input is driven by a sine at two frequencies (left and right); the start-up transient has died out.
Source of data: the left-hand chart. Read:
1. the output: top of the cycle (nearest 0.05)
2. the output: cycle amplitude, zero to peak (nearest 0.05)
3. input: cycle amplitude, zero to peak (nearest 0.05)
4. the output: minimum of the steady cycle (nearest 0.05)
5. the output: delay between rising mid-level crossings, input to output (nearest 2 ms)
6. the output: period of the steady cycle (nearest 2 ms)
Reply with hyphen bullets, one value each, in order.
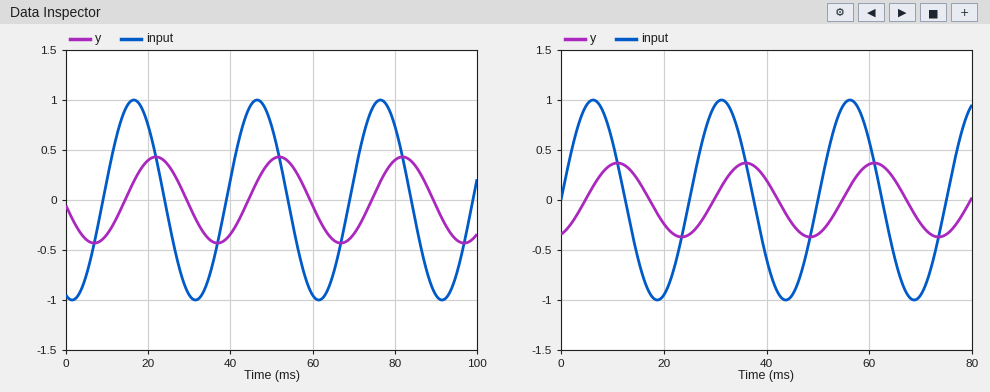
- 0.45
- 0.45
- 1.00
- -0.45
- 6 ms
- 30 ms
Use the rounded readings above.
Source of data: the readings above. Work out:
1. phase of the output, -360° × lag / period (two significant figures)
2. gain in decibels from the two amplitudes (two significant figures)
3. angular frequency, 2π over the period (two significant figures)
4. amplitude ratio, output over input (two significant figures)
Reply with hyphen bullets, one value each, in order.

- -72°
- -6.9 dB
- 0.21 rad/ms
- 0.45
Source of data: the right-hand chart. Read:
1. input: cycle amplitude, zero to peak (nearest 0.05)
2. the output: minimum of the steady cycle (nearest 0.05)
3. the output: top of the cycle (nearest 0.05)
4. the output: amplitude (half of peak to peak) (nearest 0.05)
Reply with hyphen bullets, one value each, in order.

- 1.00
- -0.35
- 0.35
- 0.35
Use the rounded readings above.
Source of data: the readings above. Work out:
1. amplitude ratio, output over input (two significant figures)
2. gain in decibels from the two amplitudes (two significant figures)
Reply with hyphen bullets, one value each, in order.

- 0.35
- -9.1 dB
